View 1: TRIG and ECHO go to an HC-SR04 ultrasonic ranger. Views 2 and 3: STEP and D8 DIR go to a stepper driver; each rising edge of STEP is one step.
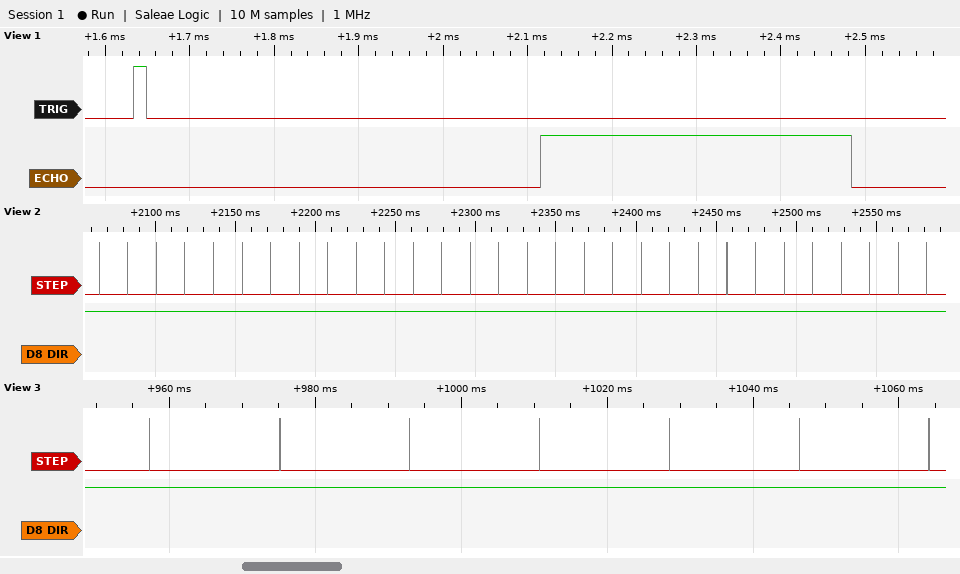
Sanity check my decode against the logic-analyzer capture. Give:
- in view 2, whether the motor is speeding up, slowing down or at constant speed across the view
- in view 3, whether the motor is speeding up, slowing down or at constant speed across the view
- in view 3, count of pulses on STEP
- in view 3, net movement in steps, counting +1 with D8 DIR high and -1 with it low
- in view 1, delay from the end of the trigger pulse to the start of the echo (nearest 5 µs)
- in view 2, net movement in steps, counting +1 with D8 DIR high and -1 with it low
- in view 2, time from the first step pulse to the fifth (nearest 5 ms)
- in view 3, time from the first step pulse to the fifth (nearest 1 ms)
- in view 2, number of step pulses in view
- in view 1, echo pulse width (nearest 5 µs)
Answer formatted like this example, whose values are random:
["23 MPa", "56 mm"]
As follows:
["constant speed", "constant speed", "7", "+7", "465 µs", "+30", "70 ms", "71 ms", "30", "370 µs"]
